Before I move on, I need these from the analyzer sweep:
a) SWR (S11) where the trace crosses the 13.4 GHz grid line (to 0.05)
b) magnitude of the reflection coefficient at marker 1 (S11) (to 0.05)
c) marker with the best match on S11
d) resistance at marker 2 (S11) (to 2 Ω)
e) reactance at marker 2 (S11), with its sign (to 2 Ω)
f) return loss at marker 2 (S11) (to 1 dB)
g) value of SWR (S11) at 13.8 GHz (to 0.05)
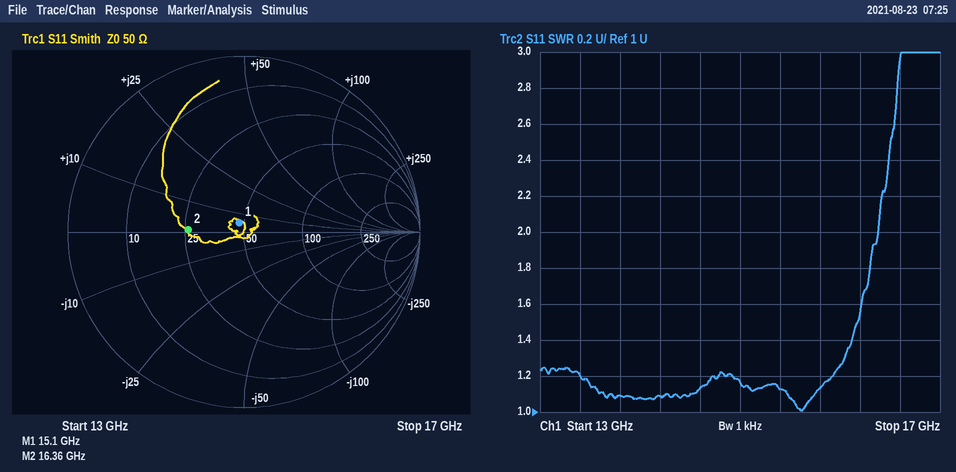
1.20
0.05
marker 1
26 Ω
0 Ω
10 dB
1.10
